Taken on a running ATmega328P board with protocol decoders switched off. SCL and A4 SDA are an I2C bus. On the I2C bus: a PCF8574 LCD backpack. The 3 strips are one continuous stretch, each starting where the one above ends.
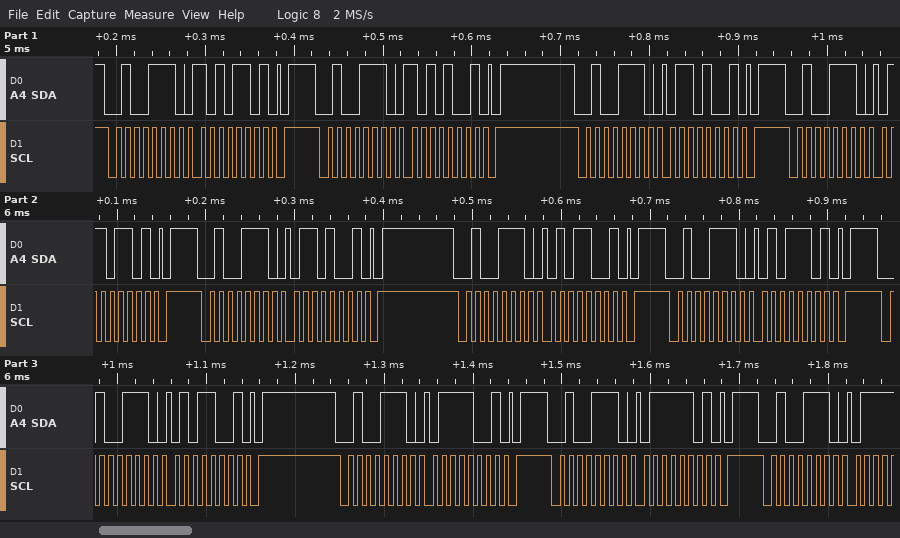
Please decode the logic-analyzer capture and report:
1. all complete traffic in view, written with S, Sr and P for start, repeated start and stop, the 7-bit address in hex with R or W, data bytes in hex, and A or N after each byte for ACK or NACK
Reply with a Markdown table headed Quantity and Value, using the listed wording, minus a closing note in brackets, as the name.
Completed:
| Quantity | Value |
|---|---|
| all complete traffic in view, written with S, Sr and P for start, repeated start and stop, the 7-bit address in hex with R or W, data bytes in hex, and A or N after each byte for ACK or NACK | S 27W A AD A P S 27W A A9 A P S 27W A 69 A P S 27W A 6D A P S 27W A 69 A P S 27W A 59 A P S 27W A 5D A P S 27W A 59 A P S 27W A 79 A P S 27W A 7D A P S 27W A |
